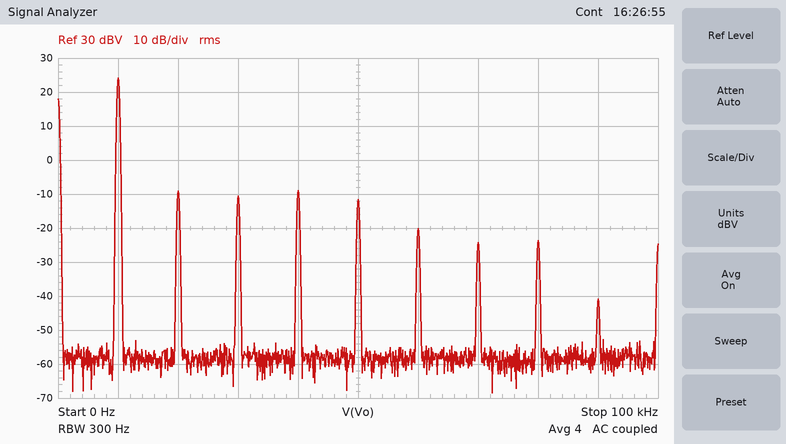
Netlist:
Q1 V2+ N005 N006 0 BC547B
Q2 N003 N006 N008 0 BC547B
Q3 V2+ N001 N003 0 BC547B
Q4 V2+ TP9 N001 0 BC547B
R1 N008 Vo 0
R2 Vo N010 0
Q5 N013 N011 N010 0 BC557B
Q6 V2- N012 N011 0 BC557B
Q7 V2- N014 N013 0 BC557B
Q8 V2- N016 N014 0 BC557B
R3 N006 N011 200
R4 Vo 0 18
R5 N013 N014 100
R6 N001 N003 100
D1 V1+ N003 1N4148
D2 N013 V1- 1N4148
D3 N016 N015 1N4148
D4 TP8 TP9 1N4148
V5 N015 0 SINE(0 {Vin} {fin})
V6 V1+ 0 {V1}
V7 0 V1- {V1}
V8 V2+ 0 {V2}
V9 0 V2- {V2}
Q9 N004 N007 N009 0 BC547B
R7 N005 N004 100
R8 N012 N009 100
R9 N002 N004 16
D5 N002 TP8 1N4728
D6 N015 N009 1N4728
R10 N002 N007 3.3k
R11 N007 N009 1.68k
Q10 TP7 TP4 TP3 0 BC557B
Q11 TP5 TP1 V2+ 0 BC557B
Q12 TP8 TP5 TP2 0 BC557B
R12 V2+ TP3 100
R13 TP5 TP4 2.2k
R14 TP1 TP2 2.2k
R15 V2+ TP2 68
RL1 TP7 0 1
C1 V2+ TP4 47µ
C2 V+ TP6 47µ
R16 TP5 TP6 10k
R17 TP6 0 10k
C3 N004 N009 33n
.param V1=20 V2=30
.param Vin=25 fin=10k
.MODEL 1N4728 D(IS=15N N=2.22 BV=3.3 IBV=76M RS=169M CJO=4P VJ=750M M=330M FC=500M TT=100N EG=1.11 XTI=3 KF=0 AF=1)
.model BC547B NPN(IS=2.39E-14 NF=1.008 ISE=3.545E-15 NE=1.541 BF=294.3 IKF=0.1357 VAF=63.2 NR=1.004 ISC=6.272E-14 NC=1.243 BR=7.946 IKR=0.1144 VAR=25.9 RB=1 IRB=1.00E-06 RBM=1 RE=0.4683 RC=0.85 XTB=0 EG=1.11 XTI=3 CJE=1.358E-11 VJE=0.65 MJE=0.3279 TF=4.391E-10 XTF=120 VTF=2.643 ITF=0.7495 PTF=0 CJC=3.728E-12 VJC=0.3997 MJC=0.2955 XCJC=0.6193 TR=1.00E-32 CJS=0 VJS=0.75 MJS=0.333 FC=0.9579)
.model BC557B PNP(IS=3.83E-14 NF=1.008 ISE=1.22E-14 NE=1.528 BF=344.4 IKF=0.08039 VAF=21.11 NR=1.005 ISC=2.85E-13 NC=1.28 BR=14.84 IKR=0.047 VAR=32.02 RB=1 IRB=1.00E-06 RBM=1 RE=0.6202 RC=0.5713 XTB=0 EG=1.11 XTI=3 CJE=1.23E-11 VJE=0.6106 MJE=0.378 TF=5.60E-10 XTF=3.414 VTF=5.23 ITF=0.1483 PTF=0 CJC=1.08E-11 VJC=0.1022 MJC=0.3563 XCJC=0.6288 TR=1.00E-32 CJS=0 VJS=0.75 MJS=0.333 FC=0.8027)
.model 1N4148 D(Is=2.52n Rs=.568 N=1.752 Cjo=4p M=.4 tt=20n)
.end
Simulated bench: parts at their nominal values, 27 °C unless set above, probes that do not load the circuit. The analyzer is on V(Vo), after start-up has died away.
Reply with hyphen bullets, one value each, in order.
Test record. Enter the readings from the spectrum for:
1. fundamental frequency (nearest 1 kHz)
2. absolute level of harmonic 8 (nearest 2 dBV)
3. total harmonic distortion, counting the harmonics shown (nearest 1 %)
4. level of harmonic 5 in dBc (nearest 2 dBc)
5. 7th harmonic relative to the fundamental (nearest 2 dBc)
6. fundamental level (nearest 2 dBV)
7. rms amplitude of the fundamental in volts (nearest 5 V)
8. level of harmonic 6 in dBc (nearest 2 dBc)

- 10 kHz
- -24 dBV
- 4 %
- -36 dBc
- -48 dBc
- 24 dBV
- 15 V
- -44 dBc
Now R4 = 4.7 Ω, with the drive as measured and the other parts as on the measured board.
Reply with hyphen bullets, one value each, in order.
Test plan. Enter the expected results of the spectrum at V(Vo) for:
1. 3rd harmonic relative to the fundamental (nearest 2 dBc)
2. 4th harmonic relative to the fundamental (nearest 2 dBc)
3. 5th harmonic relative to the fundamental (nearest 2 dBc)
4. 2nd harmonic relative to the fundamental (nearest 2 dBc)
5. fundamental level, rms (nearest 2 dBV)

- -26 dBc
- -46 dBc
- -46 dBc
- -22 dBc
- 22 dBV
